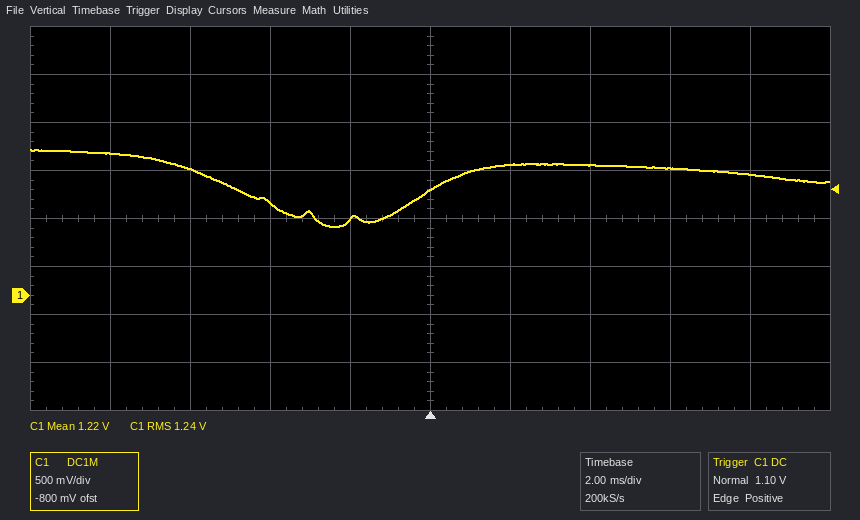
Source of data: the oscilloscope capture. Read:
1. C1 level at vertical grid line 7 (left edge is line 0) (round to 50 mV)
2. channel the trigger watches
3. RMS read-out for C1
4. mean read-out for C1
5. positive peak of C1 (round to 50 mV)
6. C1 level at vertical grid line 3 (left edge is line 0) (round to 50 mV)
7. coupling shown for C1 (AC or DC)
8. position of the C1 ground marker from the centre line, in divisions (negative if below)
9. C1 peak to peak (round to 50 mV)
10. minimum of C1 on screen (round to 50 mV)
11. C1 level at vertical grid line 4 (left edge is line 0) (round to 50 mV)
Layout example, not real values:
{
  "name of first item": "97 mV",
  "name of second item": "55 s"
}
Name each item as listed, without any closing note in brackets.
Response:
{
  "C1 level at vertical grid line 7 (left edge is line 0)": "1.35 V",
  "channel the trigger watches": "C1",
  "RMS read-out for C1": "1.24 V",
  "mean read-out for C1": "1.22 V",
  "positive peak of C1": "1.50 V",
  "C1 level at vertical grid line 3 (left edge is line 0)": "950 mV",
  "coupling shown for C1": "DC",
  "position of the C1 ground marker from the centre line, in divisions": "-1.6 div",
  "C1 peak to peak": "800 mV",
  "minimum of C1 on screen": "700 mV",
  "C1 level at vertical grid line 4 (left edge is line 0)": "800 mV"
}
